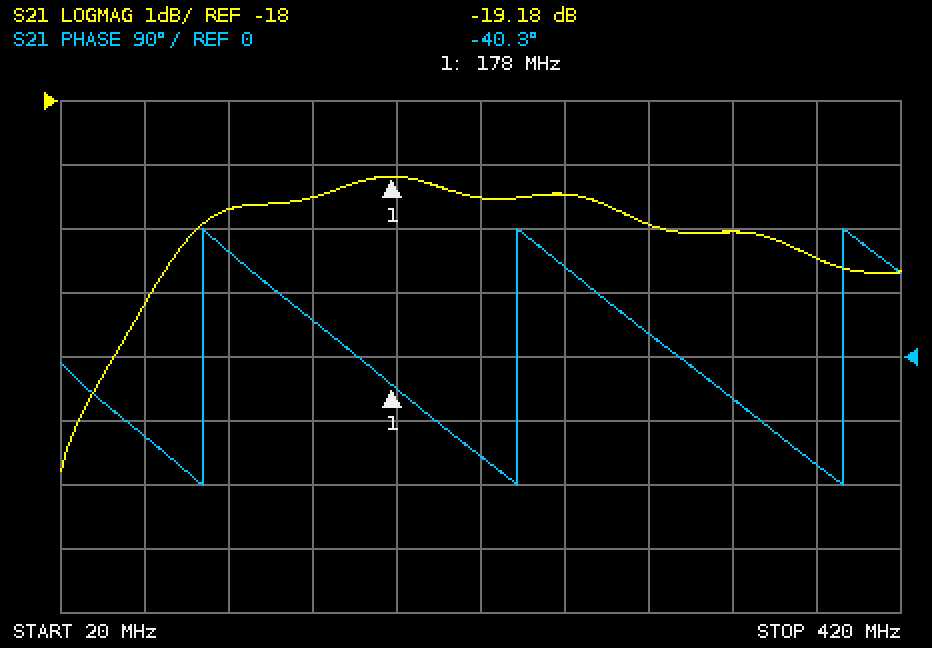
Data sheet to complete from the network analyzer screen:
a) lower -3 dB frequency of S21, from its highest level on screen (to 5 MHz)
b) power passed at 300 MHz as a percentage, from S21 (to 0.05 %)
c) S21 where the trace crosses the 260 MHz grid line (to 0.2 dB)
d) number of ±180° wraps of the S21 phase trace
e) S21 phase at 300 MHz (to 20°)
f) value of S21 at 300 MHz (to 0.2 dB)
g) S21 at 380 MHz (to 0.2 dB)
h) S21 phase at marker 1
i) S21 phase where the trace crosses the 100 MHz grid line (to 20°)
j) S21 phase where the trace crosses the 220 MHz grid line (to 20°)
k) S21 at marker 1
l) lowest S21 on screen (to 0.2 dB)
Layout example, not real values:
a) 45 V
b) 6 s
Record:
a) 40 MHz
b) 1.00 %
c) -19.4 dB
d) 3
e) 40°
f) -20.0 dB
g) -20.4 dB
h) -40.3°
i) 140°
j) -140°
k) -19.18 dB
l) -23.8 dB
